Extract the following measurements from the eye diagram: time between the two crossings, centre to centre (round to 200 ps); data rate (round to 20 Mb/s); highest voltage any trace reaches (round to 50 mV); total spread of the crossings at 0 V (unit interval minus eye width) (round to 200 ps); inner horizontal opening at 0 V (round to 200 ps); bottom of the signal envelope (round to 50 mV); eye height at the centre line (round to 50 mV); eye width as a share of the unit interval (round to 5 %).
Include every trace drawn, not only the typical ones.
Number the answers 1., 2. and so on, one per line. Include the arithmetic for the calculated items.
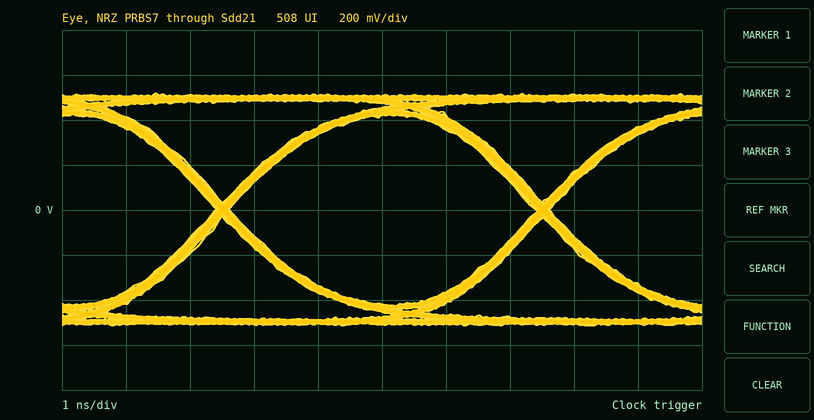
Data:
1. 5.0 ns
2. 200 Mb/s
3. 500 mV
4. 200 ps
5. 4.8 ns
6. -500 mV
7. 850 mV
8. 4.8 ns / 5.0 ns ≈ 96.0 %, so 95 % to the nearest 5 %
